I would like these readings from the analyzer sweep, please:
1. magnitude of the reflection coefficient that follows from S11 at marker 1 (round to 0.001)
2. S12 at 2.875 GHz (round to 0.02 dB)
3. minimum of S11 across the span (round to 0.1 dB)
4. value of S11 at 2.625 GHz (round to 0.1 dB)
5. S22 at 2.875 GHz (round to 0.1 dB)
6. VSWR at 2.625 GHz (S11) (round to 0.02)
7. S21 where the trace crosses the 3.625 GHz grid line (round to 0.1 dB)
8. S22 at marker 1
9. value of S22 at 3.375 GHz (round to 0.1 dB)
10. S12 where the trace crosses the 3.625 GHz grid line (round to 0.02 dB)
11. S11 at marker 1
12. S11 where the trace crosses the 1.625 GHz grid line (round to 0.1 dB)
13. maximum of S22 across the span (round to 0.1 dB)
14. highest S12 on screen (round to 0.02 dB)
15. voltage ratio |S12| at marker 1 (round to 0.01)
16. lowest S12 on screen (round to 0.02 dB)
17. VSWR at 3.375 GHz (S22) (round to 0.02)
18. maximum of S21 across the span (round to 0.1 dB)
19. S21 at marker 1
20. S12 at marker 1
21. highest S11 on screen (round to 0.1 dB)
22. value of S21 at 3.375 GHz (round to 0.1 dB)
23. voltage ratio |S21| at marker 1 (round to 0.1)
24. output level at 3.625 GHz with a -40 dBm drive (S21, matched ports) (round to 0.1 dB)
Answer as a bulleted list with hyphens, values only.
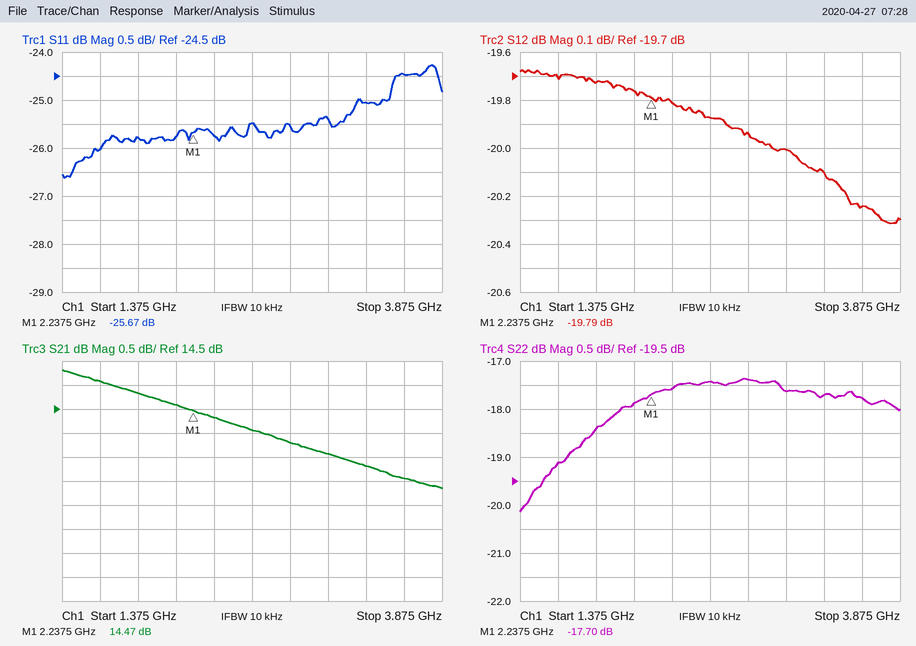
- 0.052
- -19.94 dB
- -26.6 dB
- -25.5 dB
- -17.4 dB
- 1.12
- 13.1 dB
- -17.70 dB
- -17.7 dB
- -20.24 dB
- -25.67 dB
- -26.0 dB
- -17.4 dB
- -19.68 dB
- 0.10
- -20.32 dB
- 1.30
- 15.3 dB
- 14.47 dB
- -19.79 dB
- -24.3 dB
- 13.3 dB
- 5.3
- -26.9 dBm
